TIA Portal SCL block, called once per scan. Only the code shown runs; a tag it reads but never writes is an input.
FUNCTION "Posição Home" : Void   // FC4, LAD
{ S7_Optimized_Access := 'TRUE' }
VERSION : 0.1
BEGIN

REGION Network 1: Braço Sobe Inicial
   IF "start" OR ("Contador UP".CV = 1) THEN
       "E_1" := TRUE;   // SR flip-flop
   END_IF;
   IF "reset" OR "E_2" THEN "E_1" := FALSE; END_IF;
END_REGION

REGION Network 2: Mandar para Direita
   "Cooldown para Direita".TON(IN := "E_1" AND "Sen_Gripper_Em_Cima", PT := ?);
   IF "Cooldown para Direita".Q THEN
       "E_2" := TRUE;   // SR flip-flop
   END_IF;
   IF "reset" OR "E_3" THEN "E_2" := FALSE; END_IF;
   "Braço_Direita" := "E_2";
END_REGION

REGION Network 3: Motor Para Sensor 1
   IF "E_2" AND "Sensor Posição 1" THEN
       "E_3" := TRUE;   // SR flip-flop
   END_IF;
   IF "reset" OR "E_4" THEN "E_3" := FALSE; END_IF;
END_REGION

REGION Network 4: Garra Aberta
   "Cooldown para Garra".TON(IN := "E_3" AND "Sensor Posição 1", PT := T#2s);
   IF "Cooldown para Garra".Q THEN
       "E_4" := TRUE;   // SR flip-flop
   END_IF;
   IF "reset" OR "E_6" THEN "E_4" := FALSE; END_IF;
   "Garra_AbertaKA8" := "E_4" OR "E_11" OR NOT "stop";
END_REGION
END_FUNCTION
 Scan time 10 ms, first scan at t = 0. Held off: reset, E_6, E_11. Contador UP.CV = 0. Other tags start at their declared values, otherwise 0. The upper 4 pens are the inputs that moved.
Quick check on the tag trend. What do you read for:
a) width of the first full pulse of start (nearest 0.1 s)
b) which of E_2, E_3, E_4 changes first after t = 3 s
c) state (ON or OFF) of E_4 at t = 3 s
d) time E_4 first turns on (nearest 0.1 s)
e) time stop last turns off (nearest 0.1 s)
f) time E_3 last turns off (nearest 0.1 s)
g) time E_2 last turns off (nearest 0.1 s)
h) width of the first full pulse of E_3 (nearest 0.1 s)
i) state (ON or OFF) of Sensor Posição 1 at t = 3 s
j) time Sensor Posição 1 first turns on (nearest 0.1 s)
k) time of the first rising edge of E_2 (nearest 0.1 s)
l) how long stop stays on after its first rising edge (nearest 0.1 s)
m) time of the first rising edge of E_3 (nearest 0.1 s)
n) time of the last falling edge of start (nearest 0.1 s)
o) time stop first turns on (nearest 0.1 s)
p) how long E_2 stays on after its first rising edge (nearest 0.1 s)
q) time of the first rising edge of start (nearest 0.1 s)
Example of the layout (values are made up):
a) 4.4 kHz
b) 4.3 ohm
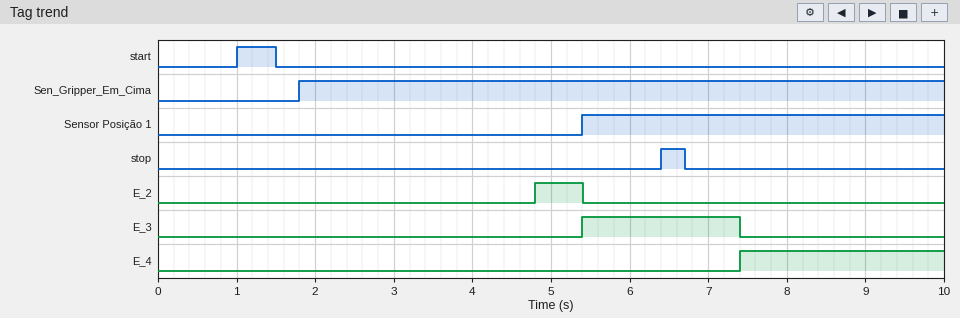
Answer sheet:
a) 0.5 s
b) E_2
c) OFF
d) 7.4 s
e) 6.7 s
f) 7.4 s
g) 5.4 s
h) 2.0 s
i) OFF
j) 5.4 s
k) 4.8 s
l) 0.3 s
m) 5.4 s
n) 1.5 s
o) 6.4 s
p) 0.6 s
q) 1.0 s
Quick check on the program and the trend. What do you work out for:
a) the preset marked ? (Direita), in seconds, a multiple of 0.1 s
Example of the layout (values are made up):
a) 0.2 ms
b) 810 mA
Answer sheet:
a) 3.0 s
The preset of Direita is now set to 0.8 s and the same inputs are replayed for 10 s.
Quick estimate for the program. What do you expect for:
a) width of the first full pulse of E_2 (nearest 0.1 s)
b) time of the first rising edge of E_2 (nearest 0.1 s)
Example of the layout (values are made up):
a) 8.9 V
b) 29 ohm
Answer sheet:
a) 2.8 s
b) 2.6 s
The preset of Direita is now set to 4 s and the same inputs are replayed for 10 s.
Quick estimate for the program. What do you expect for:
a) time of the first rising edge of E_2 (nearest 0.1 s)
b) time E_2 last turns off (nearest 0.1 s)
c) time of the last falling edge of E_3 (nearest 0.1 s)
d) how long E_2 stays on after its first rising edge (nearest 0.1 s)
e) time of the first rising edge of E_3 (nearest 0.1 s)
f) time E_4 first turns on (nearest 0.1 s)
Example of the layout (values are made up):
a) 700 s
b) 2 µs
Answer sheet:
a) 5.8 s
b) 5.8 s
c) 7.8 s
d) 0.0 s
e) 5.8 s
f) 7.8 s
